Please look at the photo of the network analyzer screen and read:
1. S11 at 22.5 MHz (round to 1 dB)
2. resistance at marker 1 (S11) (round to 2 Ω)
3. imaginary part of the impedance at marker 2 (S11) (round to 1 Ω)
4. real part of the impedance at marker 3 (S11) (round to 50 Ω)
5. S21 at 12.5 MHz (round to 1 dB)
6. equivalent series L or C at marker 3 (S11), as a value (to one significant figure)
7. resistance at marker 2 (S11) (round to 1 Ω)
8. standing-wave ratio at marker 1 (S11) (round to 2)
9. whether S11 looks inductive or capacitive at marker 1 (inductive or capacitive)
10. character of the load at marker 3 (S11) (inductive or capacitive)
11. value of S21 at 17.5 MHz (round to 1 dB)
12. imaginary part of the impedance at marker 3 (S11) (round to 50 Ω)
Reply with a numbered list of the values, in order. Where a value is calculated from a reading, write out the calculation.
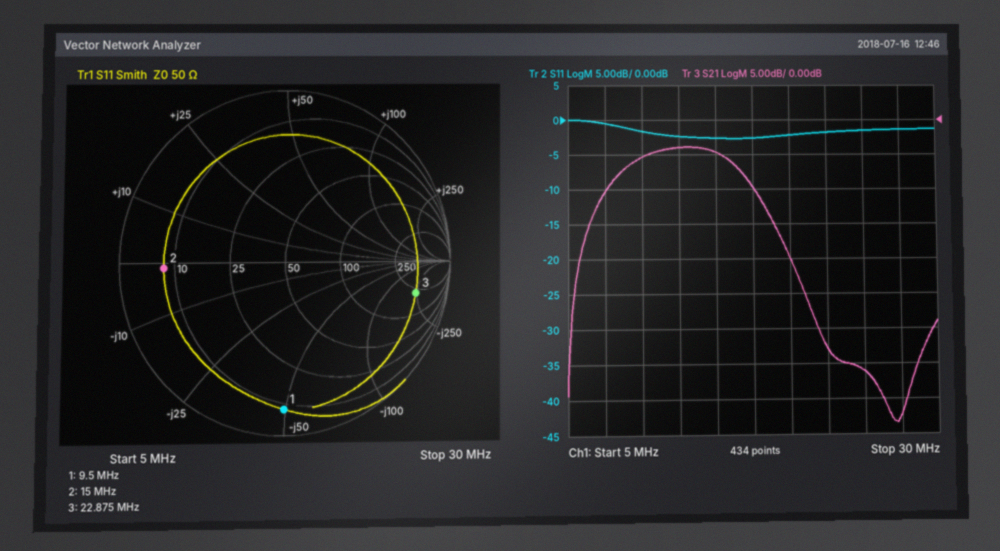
1. -2 dB
2. 8 Ω
3. -1 Ω
4. 200 Ω
5. -4 dB
6. C = 1/(2π × 22.875 MHz × 250 Ω) ≈ 27.8 pF, so 30 pF to one significant figure
7. 8 Ω
8. 12
9. capacitive
10. capacitive
11. -10 dB
12. -250 Ω
